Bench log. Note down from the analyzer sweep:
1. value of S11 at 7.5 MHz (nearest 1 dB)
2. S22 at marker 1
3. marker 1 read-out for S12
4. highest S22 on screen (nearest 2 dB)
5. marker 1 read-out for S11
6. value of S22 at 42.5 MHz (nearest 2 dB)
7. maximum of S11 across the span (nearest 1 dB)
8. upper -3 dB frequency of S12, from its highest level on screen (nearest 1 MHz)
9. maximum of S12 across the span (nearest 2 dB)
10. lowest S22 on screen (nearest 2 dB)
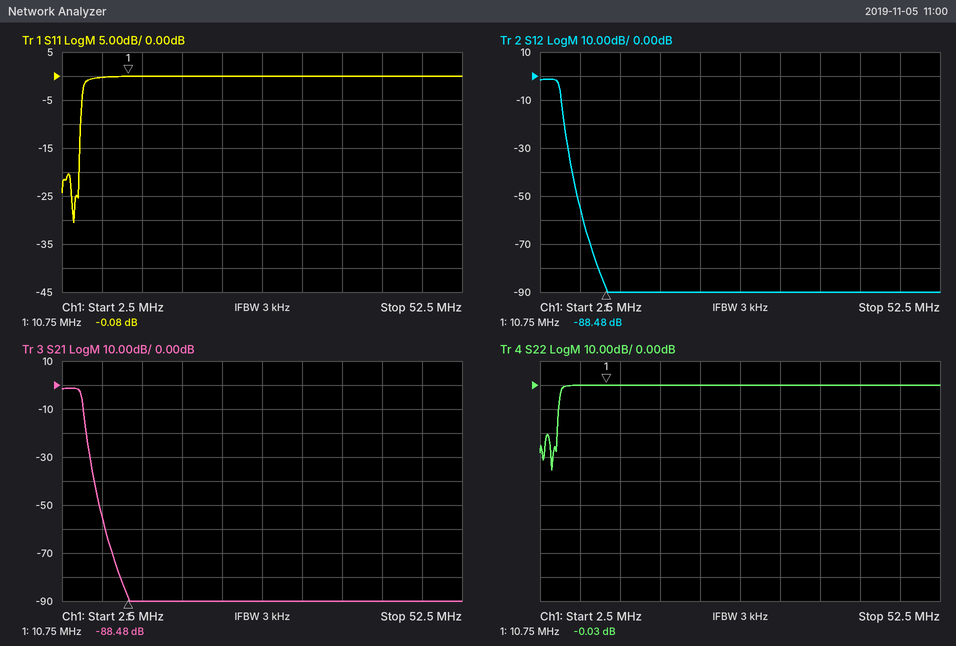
0 dB
-0.03 dB
-88.48 dB
0 dB
-0.08 dB
0 dB
0 dB
5 MHz
-2 dB
-36 dB
